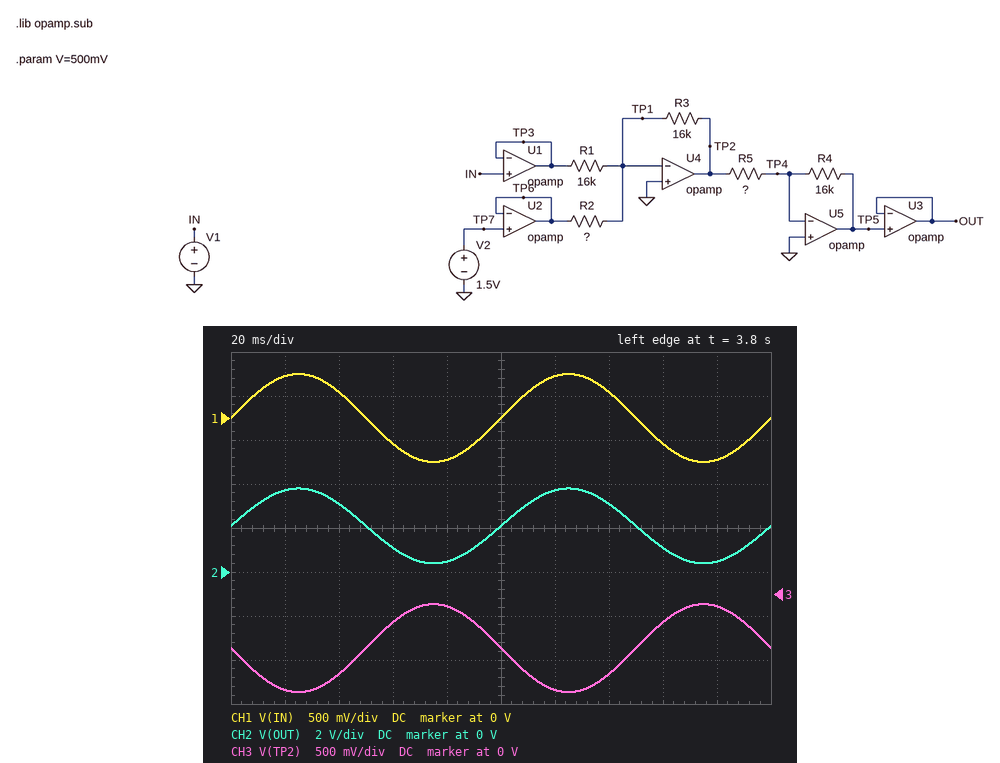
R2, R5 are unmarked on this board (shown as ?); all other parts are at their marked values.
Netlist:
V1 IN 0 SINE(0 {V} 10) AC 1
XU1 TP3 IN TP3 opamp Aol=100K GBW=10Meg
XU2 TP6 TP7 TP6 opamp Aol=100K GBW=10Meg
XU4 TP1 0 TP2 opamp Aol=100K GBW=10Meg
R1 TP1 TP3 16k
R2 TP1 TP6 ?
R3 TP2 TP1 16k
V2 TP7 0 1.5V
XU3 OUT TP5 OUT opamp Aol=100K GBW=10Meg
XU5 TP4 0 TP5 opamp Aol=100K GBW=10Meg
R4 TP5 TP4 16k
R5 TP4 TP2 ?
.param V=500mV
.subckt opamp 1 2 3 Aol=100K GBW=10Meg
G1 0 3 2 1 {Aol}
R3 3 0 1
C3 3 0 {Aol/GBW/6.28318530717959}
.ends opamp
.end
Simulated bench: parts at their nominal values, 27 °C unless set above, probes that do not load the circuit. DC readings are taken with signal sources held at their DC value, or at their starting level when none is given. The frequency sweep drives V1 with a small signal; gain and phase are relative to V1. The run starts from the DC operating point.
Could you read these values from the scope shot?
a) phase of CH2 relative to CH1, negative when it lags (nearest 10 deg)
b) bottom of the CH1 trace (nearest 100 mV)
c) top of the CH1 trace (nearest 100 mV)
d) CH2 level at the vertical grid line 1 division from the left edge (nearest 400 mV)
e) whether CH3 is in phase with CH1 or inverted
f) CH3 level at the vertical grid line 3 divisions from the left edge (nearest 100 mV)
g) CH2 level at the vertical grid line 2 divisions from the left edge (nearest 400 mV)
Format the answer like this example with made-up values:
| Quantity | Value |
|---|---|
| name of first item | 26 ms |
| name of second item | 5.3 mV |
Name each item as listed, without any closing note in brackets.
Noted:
| Quantity | Value |
|---|---|
| phase of CH2 relative to CH1, negative when it lags | 0 deg |
| bottom of the CH1 trace | -500 mV |
| top of the CH1 trace | 500 mV |
| CH2 level at the vertical grid line 1 division from the left edge | 3.6 V |
| whether CH3 is in phase with CH1 or inverted | inverted |
| CH3 level at the vertical grid line 3 divisions from the left edge | -300 mV |
| CH2 level at the vertical grid line 2 divisions from the left edge | 3.2 V |
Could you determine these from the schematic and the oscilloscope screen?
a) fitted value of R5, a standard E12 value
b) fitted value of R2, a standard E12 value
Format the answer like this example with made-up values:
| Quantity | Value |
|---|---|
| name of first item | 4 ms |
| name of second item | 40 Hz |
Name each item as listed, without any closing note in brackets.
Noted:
| Quantity | Value |
|---|---|
| fitted value of R5, a standard E12 value | 4.7 kΩ |
| fitted value of R2, a standard E12 value | 39 kΩ |
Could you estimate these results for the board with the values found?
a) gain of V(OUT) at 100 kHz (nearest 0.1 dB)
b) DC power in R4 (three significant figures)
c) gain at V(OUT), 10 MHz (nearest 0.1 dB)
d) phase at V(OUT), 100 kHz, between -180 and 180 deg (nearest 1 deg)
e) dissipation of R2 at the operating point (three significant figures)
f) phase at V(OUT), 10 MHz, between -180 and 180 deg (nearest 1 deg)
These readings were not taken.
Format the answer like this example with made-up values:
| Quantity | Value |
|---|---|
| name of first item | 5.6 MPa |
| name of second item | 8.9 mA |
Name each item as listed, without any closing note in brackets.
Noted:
| Quantity | Value |
|---|---|
| gain of V(OUT) at 100 kHz | 10.6 dB |
| DC power in R4 | 274 µW |
| gain at V(OUT), 10 MHz | -16.8 dB |
| phase at V(OUT), 100 kHz, between -180 and 180 deg | -5 deg |
| dissipation of R2 at the operating point | 57.7 µW |
| phase at V(OUT), 10 MHz, between -180 and 180 deg | 125 deg |
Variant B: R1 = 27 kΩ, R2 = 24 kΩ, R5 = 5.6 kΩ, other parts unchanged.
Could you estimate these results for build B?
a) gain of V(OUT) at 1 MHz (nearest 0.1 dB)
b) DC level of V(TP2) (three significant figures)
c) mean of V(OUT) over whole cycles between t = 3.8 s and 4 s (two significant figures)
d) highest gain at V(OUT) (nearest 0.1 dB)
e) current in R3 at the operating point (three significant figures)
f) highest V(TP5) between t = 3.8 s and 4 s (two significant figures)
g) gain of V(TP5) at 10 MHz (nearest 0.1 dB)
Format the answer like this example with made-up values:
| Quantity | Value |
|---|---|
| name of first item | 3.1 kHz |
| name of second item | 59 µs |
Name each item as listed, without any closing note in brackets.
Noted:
| Quantity | Value |
|---|---|
| gain of V(OUT) at 1 MHz | 3.7 dB |
| DC level of V(TP2) | -1.00 V |
| mean of V(OUT) over whole cycles between t = 3.8 s and 4 s | 2.9 V |
| highest gain at V(OUT) | 4.6 dB |
| current in R3 at the operating point | 62.5 µA |
| highest V(TP5) between t = 3.8 s and 4 s | 3.7 V |
| gain of V(TP5) at 10 MHz | -18.3 dB |
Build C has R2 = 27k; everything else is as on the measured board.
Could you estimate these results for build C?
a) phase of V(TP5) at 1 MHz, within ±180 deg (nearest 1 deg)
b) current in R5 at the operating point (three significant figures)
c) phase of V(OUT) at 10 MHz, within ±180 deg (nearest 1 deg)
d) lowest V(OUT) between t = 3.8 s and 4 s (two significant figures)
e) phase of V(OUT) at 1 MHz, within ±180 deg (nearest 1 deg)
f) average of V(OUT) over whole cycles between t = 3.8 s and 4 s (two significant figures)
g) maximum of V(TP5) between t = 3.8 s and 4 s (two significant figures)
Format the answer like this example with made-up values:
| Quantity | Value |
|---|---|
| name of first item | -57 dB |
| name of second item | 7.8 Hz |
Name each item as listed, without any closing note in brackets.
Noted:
| Quantity | Value |
|---|---|
| phase of V(TP5) at 1 MHz, within ±180 deg | -44 deg |
| current in R5 at the operating point | 189 µA |
| phase of V(OUT) at 10 MHz, within ±180 deg | 124 deg |
| lowest V(OUT) between t = 3.8 s and 4 s | 1.3 V |
| phase of V(OUT) at 1 MHz, within ±180 deg | -50 deg |
| average of V(OUT) over whole cycles between t = 3.8 s and 4 s | 3.0 V |
| maximum of V(TP5) between t = 3.8 s and 4 s | 4.7 V |
